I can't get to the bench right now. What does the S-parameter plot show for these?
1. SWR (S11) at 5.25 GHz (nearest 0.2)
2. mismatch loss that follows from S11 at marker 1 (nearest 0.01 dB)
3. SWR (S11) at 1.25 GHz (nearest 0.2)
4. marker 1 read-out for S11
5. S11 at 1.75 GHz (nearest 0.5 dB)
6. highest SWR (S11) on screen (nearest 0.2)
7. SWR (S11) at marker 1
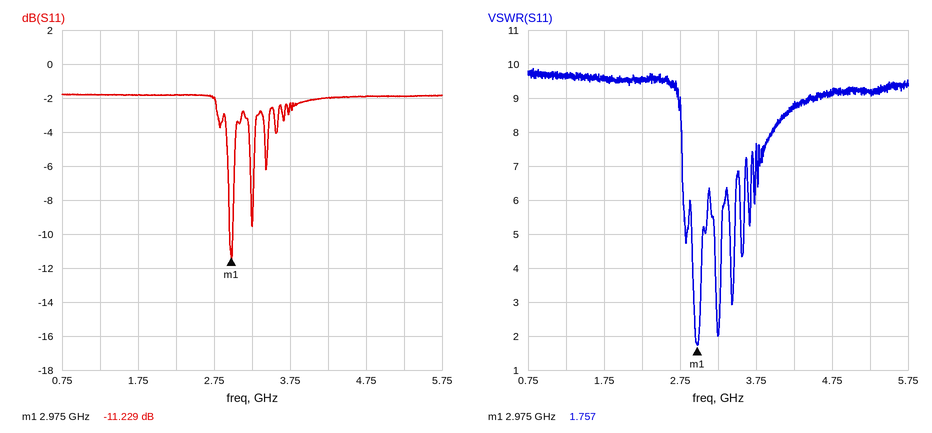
9.2
0.34 dB
9.6
-11.229 dB
-2.0 dB
9.8
1.757
